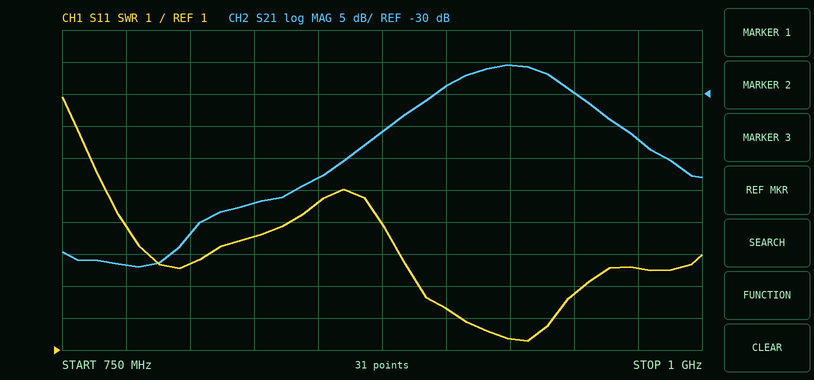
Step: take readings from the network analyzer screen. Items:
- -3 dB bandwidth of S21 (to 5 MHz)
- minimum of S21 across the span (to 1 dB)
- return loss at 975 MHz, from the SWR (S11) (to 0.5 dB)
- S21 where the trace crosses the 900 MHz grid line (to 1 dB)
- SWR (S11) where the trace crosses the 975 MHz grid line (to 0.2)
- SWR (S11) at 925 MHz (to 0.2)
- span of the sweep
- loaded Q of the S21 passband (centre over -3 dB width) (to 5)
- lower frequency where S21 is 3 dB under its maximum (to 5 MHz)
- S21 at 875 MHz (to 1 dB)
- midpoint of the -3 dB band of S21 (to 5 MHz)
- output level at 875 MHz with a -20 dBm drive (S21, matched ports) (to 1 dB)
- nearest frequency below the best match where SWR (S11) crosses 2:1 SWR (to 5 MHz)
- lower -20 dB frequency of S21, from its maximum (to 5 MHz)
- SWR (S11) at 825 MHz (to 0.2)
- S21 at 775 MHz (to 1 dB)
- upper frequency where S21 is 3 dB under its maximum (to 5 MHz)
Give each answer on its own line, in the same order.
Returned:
45 MHz
-57 dB
5.0 dB
-29 dB
3.6
1.4
250 MHz
20
900 MHz
-36 dB
925 MHz
-56 dBm
905 MHz
840 MHz
4.6
-57 dB
945 MHz
